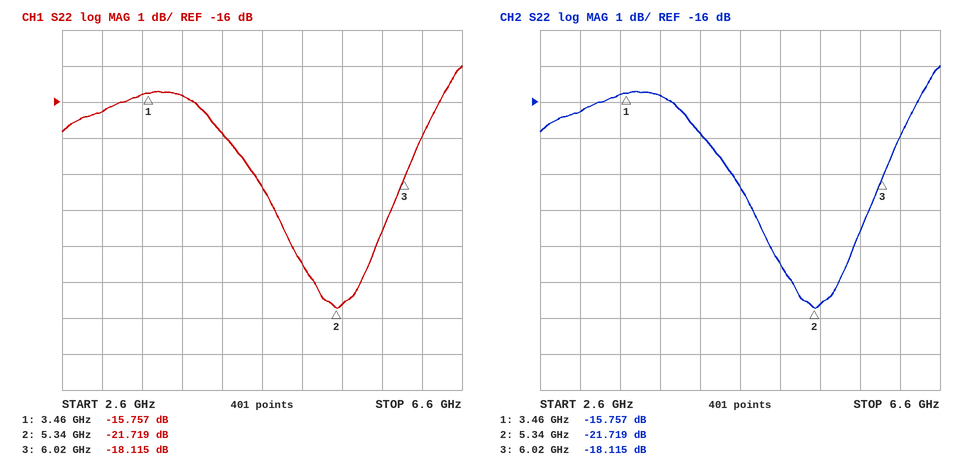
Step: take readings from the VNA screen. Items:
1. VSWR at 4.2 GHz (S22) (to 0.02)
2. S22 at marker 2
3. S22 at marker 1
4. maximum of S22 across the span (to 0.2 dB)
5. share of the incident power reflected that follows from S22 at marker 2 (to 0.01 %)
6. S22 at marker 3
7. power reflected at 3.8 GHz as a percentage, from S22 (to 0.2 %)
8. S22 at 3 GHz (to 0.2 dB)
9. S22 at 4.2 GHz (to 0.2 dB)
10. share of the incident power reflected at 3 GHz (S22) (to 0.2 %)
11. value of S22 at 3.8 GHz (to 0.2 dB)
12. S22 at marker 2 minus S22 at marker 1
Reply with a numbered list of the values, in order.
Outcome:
1. 1.34
2. -21.719 dB
3. -15.757 dB
4. -15.0 dB
5. 0.67 %
6. -18.115 dB
7. 2.6 %
8. -16.2 dB
9. -16.8 dB
10. 2.4 %
11. -15.8 dB
12. -5.962 dB
